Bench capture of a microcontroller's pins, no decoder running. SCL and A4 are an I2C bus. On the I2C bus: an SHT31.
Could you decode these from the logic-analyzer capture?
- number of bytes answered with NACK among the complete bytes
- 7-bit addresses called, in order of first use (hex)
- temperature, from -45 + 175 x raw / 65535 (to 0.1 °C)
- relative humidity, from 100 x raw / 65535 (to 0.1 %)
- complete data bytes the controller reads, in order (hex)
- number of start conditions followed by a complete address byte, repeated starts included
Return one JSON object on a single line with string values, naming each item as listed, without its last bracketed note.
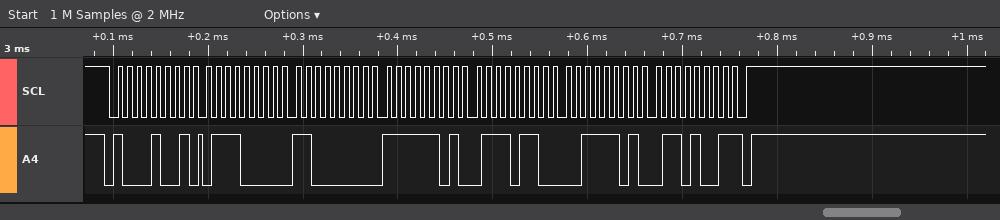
{"number of bytes answered with NACK among the complete bytes": "1", "7-bit addresses called, in order of first use": "0x44", "temperature, from -45 + 175 x raw / 65535": "32.1 °C", "relative humidity, from 100 x raw / 65535": "46.2 %", "complete data bytes the controller reads, in order": "70 C0 FD 76 3D 69", "number of start conditions followed by a complete address byte, repeated starts included": "1"}
